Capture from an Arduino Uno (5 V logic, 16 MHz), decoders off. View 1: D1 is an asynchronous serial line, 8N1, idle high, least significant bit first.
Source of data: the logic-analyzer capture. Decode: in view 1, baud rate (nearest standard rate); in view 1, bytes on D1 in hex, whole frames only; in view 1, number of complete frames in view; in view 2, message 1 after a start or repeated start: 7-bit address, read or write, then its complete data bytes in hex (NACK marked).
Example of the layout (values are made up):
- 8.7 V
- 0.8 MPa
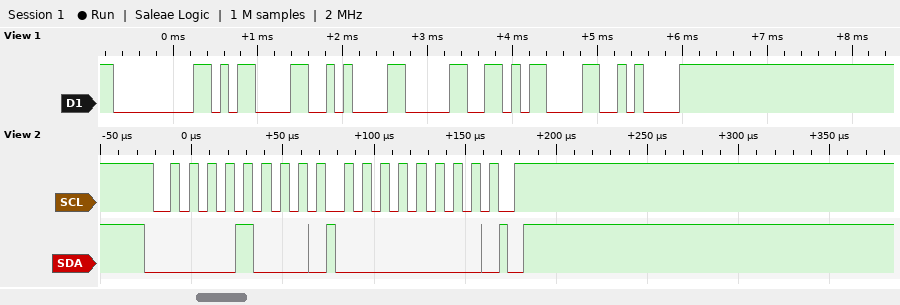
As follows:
- 9600 baud
- 0x00 0x0D 0x0A 0x30 0x0D 0x0A
- 6
- 0x04 write: 00
